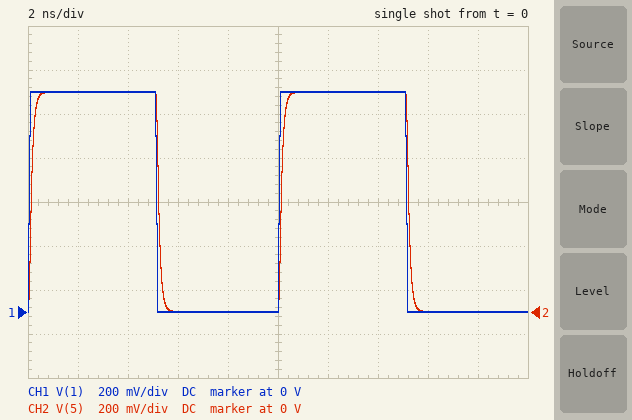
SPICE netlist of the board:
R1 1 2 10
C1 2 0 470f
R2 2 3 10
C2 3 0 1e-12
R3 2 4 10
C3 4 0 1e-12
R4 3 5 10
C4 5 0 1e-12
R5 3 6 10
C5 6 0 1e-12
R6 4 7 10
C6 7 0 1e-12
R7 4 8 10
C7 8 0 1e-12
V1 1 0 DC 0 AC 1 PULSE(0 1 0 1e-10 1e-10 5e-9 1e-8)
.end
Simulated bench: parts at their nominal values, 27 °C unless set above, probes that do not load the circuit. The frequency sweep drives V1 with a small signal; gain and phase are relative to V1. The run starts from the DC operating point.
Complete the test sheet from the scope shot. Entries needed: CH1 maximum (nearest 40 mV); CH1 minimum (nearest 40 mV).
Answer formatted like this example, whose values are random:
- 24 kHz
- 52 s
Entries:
- 1.00 V
- 0 V
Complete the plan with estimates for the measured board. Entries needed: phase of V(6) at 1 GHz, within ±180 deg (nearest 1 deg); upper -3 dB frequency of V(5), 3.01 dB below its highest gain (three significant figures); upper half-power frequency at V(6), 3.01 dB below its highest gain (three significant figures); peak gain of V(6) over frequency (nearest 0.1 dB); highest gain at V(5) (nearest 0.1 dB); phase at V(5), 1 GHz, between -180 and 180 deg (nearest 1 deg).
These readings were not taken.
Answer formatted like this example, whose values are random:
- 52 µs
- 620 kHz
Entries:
- -34 deg
- 1.59 GHz
- 1.59 GHz
- 0 dB
- 0 dB
- -34 deg
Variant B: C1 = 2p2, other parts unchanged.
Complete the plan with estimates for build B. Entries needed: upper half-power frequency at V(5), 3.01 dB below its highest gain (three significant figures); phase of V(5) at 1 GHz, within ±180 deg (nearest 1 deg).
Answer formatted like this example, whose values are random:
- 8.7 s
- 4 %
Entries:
- 1.42 GHz
- -39 deg
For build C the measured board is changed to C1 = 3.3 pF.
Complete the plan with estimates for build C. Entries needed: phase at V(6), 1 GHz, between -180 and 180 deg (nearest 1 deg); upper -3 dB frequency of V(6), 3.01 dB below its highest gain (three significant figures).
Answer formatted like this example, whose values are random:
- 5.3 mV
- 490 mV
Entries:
- -42 deg
- 1.32 GHz
